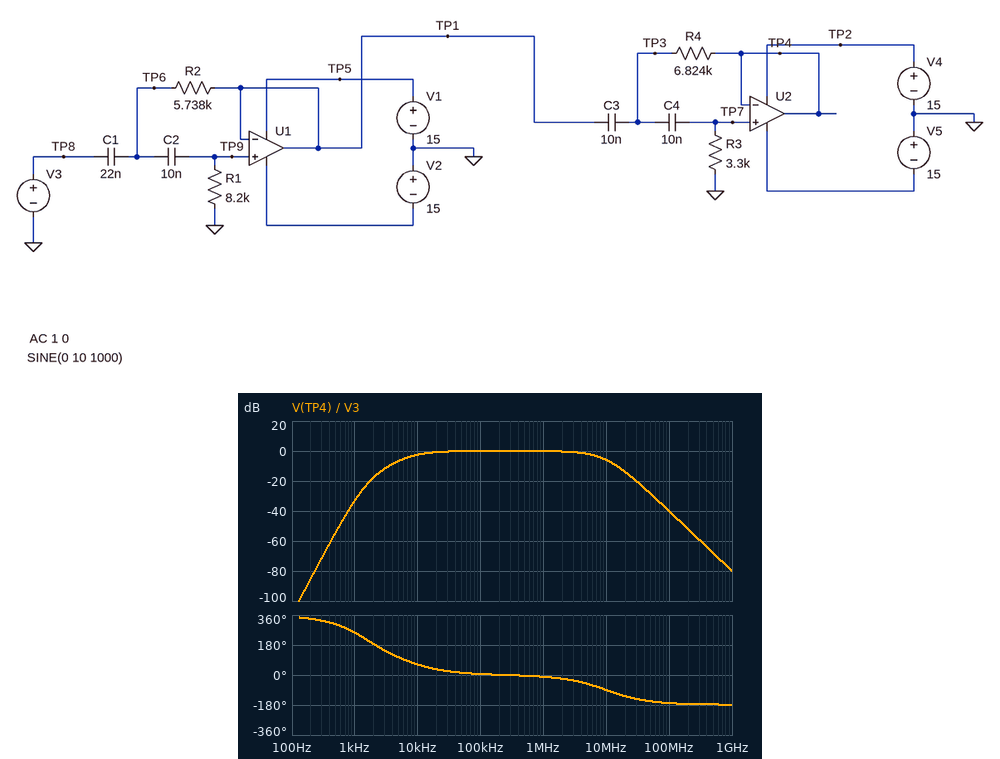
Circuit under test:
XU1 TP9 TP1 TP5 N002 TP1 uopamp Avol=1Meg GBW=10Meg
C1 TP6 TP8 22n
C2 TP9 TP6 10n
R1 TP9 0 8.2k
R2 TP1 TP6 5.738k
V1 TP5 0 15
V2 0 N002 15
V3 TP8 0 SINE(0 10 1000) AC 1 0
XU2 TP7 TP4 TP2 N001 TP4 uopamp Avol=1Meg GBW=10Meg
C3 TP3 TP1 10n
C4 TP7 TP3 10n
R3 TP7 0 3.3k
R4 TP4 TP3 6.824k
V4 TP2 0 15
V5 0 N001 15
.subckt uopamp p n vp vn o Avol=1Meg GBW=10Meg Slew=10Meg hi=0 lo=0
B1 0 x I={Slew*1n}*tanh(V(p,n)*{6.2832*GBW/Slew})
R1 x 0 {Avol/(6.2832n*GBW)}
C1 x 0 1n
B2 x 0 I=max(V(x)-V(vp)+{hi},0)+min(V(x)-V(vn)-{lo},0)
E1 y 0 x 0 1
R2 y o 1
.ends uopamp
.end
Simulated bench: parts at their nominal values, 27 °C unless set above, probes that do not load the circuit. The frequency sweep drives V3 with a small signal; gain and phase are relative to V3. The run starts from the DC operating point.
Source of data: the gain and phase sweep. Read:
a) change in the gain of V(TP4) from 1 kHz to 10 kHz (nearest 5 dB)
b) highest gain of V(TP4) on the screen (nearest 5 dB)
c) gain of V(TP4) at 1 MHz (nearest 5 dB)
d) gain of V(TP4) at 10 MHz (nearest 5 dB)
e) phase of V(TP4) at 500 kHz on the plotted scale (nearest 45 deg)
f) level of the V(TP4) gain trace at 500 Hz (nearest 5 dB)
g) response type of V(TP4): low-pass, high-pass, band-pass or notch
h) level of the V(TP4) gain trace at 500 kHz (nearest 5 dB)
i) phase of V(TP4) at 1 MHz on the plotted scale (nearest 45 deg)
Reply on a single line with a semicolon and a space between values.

30 dB; 0 dB; 0 dB; -5 dB; 0 deg; -55 dB; band-pass; 0 dB; 0 deg
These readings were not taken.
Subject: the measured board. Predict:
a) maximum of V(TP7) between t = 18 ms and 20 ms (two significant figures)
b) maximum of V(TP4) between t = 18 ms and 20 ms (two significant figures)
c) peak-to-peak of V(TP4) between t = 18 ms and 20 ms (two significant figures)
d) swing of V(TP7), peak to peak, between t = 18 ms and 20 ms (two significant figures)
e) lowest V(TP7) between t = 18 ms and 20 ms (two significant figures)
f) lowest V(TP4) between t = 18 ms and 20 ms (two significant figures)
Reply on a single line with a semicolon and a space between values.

220 mV; 220 mV; 450 mV; 450 mV; -220 mV; -220 mV
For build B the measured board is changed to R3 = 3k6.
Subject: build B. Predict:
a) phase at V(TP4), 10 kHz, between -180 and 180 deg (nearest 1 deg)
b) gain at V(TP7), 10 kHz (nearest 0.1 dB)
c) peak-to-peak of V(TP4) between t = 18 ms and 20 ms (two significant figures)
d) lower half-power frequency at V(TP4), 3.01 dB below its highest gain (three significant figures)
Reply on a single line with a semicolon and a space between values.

61 deg; -2.1 dB; 490 mV; 8.06 kHz
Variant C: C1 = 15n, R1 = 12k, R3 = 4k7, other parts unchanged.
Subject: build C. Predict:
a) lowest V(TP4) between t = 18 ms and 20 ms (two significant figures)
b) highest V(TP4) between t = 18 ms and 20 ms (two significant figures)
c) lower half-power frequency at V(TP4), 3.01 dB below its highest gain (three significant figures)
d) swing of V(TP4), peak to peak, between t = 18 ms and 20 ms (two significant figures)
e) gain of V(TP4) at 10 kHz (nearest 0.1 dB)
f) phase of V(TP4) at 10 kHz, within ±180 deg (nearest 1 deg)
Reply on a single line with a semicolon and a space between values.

-390 mV; 390 mV; 5.68 kHz; 780 mV; -1.2 dB; 49 deg
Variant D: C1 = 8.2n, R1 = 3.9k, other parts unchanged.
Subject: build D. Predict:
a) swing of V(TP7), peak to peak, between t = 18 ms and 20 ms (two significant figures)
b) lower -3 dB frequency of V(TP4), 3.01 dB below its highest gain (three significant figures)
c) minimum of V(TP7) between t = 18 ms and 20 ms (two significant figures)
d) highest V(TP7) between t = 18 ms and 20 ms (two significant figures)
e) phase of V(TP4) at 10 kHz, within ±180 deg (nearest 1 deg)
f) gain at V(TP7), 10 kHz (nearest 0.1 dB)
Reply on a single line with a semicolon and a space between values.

91 mV; 12.3 kHz; -45 mV; 45 mV; 94 deg; -4.3 dB
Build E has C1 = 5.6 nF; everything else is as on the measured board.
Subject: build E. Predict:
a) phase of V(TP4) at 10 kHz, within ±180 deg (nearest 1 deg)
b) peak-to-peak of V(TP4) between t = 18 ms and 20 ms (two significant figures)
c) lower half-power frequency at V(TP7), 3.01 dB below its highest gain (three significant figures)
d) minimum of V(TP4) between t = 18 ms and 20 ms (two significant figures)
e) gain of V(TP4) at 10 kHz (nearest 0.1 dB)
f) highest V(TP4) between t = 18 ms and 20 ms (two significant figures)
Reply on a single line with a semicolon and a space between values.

78 deg; 140 mV; 9.55 kHz; -70 mV; -2.8 dB; 70 mV
